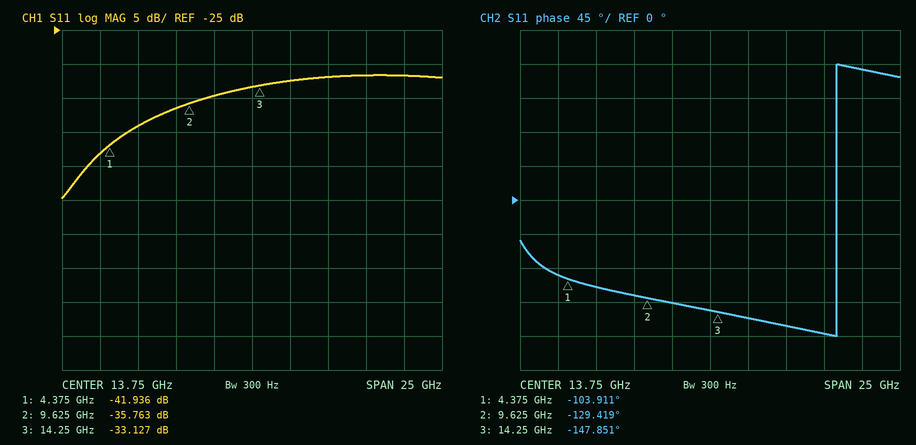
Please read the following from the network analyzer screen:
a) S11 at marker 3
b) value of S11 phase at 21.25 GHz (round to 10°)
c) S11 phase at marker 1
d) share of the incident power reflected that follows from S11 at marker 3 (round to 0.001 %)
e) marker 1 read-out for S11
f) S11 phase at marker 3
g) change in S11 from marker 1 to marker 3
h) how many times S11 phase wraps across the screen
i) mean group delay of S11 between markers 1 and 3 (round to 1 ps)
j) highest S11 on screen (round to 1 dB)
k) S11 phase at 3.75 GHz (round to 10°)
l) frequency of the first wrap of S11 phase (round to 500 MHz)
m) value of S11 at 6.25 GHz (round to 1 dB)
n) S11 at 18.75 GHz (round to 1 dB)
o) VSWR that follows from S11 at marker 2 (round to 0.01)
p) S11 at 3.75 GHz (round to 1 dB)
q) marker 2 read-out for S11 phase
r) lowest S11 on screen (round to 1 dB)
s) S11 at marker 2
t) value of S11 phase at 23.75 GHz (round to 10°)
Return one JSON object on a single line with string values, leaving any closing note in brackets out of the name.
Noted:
{"S11 at marker 3": "-33.127 dB", "value of S11 phase at 21.25 GHz": "-180°", "S11 phase at marker 1": "-103.911°", "share of the incident power reflected that follows from S11 at marker 3": "0.049 %", "marker 1 read-out for S11": "-41.936 dB", "S11 phase at marker 3": "-147.851°", "change in S11 from marker 1 to marker 3": "8.809 dB", "how many times S11 phase wraps across the screen": "1", "mean group delay of S11 between markers 1 and 3": "12 ps", "highest S11 on screen": "-32 dB", "S11 phase at 3.75 GHz": "-100°", "frequency of the first wrap of S11 phase": "22.0 GHz", "value of S11 at 6.25 GHz": "-39 dB", "S11 at 18.75 GHz": "-32 dB", "VSWR that follows from S11 at marker 2": "1.03", "S11 at 3.75 GHz": "-43 dB", "marker 2 read-out for S11 phase": "-129.419°", "lowest S11 on screen": "-50 dB", "S11 at marker 2": "-35.763 dB", "value of S11 phase at 23.75 GHz": "170°"}
